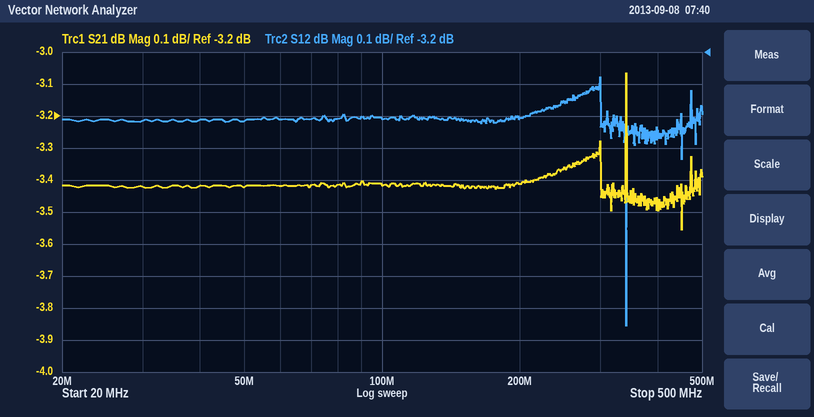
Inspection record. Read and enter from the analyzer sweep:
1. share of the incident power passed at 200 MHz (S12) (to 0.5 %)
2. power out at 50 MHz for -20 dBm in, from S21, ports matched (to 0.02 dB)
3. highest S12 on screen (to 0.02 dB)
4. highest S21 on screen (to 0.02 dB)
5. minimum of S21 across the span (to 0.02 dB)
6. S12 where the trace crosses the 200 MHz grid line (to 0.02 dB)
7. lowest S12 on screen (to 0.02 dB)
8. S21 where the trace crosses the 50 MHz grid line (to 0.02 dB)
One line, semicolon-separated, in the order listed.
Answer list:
45.5 %; -23.42 dBm; -3.28 dB; -3.06 dB; -3.56 dB; -3.40 dB; -4.06 dB; -3.42 dB
